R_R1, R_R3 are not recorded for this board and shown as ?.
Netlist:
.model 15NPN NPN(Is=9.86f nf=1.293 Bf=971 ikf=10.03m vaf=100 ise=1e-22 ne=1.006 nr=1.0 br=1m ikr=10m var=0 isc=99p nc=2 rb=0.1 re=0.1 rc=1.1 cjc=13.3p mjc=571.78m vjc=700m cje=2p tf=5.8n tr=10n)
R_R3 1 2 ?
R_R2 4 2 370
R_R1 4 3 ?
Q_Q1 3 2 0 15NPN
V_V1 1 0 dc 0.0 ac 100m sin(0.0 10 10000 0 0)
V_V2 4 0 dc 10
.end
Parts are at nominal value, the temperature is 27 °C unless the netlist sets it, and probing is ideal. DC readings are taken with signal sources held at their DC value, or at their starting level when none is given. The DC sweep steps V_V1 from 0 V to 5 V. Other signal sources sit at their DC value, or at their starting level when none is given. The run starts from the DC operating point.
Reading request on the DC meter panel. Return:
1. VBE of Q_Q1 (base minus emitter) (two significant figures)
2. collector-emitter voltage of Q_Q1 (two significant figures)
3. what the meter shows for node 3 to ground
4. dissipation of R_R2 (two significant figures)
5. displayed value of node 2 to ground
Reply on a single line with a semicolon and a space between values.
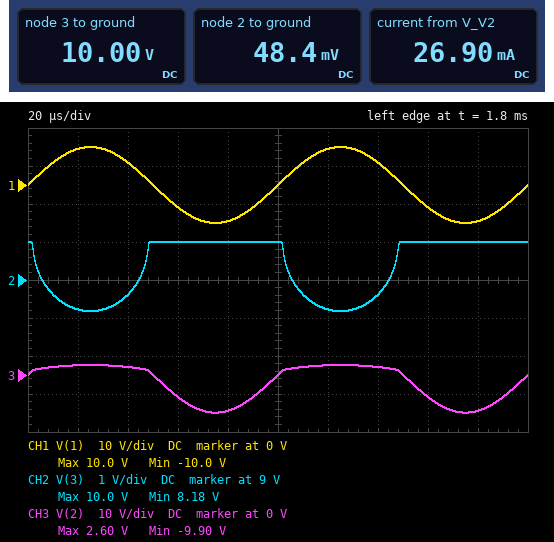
48 mV; 10 V; 10.00 V; 270 mW; 48.4 mV
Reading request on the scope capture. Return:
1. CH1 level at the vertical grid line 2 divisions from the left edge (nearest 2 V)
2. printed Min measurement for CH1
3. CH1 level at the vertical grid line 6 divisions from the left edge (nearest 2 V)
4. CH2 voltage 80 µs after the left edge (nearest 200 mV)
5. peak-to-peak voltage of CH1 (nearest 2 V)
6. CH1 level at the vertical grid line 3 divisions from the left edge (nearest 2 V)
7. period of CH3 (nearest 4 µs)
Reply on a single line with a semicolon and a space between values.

6 V; -10.0 V; 10 V; 10.0 V; 20 V; -6 V; 100 µs
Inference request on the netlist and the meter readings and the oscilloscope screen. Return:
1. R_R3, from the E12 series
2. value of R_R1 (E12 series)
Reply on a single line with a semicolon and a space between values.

1.8 Ω; 0.39 Ω
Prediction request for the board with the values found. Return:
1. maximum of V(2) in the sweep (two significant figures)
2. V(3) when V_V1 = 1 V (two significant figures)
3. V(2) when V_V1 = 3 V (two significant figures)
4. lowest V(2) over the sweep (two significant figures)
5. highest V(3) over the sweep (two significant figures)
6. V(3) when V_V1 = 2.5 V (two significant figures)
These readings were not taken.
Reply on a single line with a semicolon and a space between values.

2.0 V; 10 V; 1.7 V; 48 mV; 10 V; 9.2 V
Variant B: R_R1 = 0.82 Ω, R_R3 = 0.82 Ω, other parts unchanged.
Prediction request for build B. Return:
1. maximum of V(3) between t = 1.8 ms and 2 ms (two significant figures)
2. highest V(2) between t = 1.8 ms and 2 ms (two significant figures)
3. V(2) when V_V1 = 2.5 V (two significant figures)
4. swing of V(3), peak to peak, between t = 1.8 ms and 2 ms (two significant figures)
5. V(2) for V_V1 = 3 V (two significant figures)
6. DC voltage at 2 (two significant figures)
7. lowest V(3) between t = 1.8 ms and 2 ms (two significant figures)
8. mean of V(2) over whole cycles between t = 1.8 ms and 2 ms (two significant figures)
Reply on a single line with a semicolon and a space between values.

10 V; 3.4 V; 1.7 V; 3.6 V; 1.9 V; 22 mV; 6.4 V; -1.9 V
